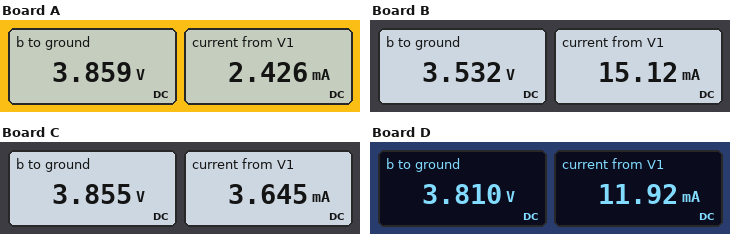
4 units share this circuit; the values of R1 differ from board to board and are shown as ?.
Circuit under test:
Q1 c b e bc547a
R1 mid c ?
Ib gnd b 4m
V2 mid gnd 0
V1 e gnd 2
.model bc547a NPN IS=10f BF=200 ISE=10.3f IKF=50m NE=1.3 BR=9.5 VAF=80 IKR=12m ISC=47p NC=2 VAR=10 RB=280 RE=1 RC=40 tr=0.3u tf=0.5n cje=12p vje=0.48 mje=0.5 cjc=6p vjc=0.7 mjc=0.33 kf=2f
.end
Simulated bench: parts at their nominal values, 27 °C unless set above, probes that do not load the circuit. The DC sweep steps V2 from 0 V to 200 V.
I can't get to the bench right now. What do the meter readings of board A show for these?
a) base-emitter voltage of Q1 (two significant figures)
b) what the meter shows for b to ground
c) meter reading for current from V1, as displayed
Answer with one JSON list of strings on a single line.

["1.9 V", "3.859 V", "2.426 mA"]
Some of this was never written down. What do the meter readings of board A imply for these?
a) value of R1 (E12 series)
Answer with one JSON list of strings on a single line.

["270 Ω"]
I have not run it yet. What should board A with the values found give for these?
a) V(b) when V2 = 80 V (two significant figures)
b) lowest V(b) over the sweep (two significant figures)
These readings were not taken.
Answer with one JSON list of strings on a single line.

["4.1 V", "3.9 V"]
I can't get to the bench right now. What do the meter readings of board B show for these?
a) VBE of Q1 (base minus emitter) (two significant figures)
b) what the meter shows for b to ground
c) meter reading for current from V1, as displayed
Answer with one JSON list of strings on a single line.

["1.5 V", "3.532 V", "15.12 mA"]
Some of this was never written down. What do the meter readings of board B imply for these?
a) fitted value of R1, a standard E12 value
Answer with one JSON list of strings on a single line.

["47 Ω"]
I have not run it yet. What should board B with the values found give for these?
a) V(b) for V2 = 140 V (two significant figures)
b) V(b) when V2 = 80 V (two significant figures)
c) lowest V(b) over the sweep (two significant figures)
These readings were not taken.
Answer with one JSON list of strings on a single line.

["4.3 V", "4.2 V", "3.5 V"]
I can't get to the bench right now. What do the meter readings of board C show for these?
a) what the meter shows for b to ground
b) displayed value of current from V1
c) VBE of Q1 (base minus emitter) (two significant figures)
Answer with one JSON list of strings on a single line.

["3.855 V", "3.645 mA", "1.9 V"]
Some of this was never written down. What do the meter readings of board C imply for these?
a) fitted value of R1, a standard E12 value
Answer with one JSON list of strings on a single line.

["220 Ω"]
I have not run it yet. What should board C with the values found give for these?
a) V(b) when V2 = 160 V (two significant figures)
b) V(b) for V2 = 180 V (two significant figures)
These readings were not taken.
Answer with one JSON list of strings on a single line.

["4.3 V", "4.3 V"]
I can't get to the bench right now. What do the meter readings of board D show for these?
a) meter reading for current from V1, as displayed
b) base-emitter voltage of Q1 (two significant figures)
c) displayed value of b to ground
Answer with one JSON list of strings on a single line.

["11.92 mA", "1.8 V", "3.810 V"]
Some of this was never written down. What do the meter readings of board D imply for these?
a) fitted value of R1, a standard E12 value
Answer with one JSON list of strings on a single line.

["82 Ω"]
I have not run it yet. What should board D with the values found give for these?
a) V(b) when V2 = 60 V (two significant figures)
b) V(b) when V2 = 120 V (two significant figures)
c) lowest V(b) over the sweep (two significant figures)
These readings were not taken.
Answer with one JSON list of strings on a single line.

["4.2 V", "4.3 V", "3.8 V"]
